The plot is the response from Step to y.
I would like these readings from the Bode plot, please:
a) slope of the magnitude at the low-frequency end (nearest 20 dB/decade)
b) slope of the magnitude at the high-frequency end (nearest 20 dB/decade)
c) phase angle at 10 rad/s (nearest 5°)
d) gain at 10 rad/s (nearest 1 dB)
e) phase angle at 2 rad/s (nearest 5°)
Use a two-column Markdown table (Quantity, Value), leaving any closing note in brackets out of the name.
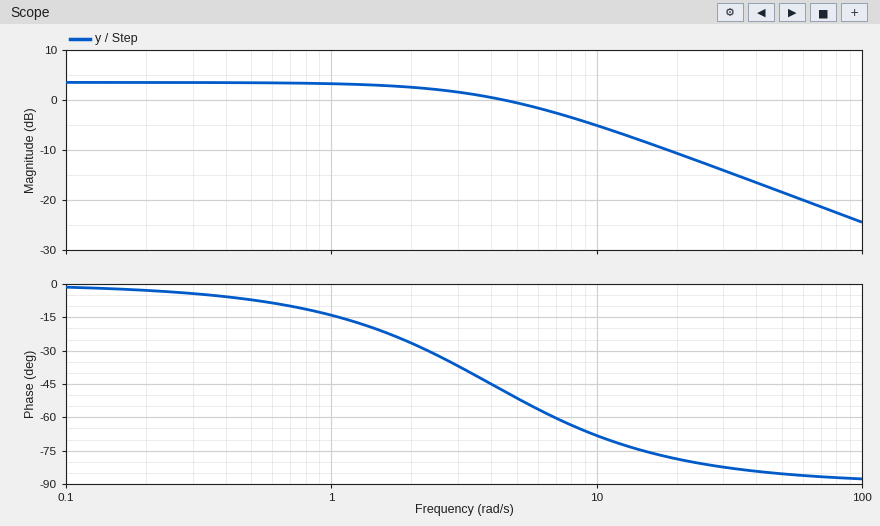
| Quantity | Value |
|---|---|
| slope of the magnitude at the low-frequency end | 0 dB/decade |
| slope of the magnitude at the high-frequency end | -20 dB/decade |
| phase angle at 10 rad/s | -70° |
| gain at 10 rad/s | -5 dB |
| phase angle at 2 rad/s | -25° |
